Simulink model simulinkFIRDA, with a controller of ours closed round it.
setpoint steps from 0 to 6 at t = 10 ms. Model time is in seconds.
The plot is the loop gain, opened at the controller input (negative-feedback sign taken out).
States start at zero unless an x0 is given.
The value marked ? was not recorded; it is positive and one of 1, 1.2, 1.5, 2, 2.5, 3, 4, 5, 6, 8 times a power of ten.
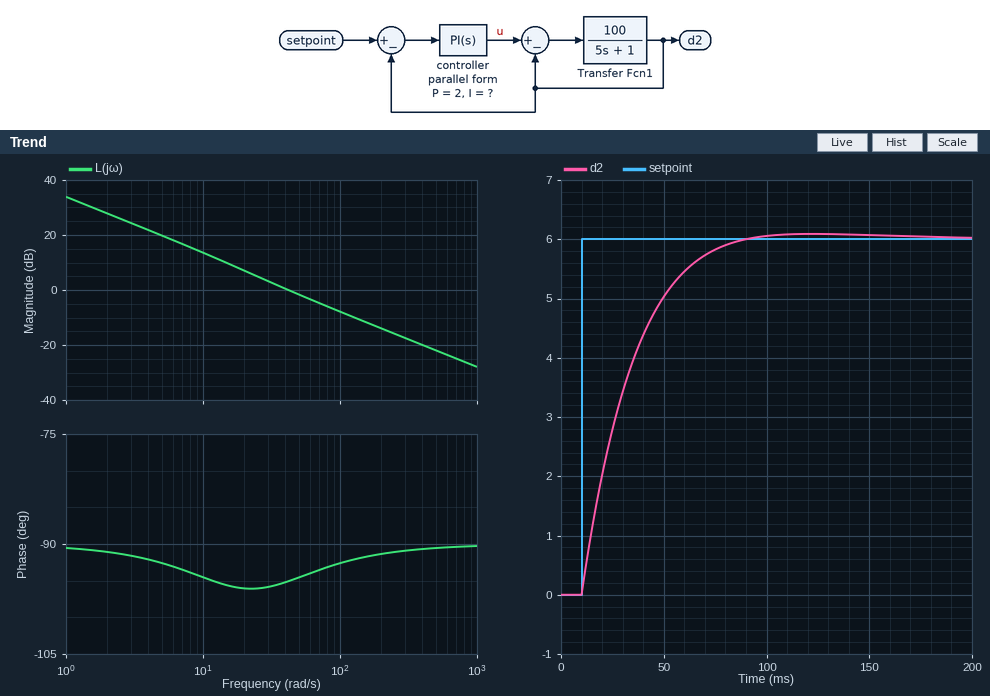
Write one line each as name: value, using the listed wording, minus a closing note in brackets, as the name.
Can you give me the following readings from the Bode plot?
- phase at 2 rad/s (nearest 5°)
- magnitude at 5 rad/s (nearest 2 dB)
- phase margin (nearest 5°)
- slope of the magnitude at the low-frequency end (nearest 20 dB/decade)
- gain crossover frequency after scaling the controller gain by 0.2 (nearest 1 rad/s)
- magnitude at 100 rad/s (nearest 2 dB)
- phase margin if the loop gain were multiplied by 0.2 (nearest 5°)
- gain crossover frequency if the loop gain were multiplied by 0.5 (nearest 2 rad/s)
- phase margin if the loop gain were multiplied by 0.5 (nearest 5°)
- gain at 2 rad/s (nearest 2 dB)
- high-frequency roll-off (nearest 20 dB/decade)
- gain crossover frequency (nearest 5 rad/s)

phase at 2 rad/s: -90°
magnitude at 5 rad/s: 20 dB
phase margin: 85°
slope of the magnitude at the low-frequency end: -20 dB/decade
gain crossover frequency after scaling the controller gain by 0.2: 10 rad/s
magnitude at 100 rad/s: -8 dB
phase margin if the loop gain were multiplied by 0.2: 85°
gain crossover frequency if the loop gain were multiplied by 0.5: 22 rad/s
phase margin if the loop gain were multiplied by 0.5: 85°
gain at 2 rad/s: 28 dB
high-frequency roll-off: -20 dB/decade
gain crossover frequency: 40 rad/s
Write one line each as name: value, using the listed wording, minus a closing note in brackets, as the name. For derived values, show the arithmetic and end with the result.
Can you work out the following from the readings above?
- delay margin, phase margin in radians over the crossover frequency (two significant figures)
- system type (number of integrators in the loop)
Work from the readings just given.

delay margin, phase margin in radians over the crossover frequency: 85 × π / 180 / 40 = 0.037 s
system type: 1
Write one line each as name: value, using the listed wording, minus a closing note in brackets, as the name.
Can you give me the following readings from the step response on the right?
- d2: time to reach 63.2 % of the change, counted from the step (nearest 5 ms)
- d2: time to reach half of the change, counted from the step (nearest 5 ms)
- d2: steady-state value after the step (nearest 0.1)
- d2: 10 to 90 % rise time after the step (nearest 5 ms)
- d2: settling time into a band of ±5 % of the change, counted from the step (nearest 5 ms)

d2: time to reach 63.2 % of the change, counted from the step: 25 ms
d2: time to reach half of the change, counted from the step: 15 ms
d2: steady-state value after the step: 6.0
d2: 10 to 90 % rise time after the step: 45 ms
d2: settling time into a band of ±5 % of the change, counted from the step: 60 ms
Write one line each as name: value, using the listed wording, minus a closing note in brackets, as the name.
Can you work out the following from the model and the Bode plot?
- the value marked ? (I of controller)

the value marked ?: 50
